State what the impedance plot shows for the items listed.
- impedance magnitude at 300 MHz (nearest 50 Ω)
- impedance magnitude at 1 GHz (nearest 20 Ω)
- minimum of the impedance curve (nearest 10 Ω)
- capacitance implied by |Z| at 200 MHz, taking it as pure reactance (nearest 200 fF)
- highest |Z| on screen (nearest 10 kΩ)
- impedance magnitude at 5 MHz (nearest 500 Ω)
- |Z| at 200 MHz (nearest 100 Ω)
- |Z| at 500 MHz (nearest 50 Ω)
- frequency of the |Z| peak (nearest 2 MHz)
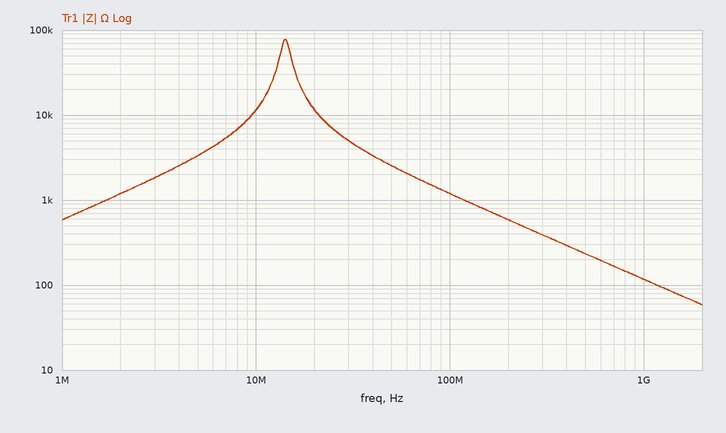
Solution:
400 Ω
120 Ω
60 Ω
1.4 pF
80 kΩ
3.5 kΩ
600 Ω
250 Ω
14 MHz
